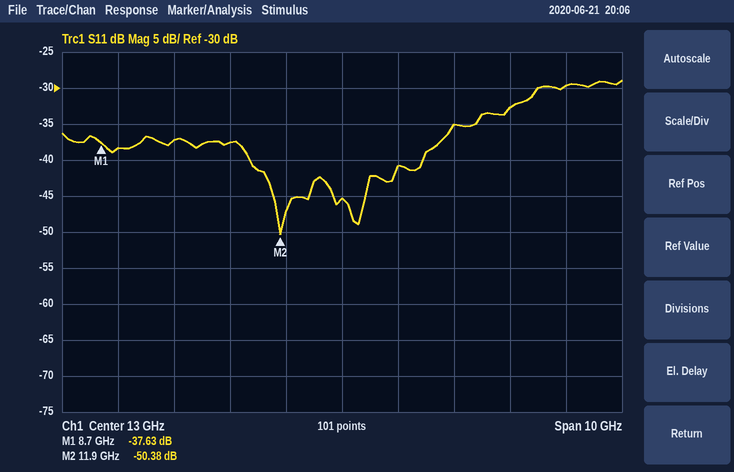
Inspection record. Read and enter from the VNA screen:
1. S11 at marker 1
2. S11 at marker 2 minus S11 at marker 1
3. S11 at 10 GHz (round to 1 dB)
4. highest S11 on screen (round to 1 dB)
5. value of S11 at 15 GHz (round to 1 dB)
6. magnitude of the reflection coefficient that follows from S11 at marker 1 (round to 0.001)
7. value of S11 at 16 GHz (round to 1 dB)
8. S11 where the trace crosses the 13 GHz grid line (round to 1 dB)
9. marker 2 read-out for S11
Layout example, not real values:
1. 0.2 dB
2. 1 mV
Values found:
1. -37.63 dB
2. -12.75 dB
3. -37 dB
4. -29 dB
5. -35 dB
6. 0.013
7. -33 dB
8. -45 dB
9. -50.38 dB
